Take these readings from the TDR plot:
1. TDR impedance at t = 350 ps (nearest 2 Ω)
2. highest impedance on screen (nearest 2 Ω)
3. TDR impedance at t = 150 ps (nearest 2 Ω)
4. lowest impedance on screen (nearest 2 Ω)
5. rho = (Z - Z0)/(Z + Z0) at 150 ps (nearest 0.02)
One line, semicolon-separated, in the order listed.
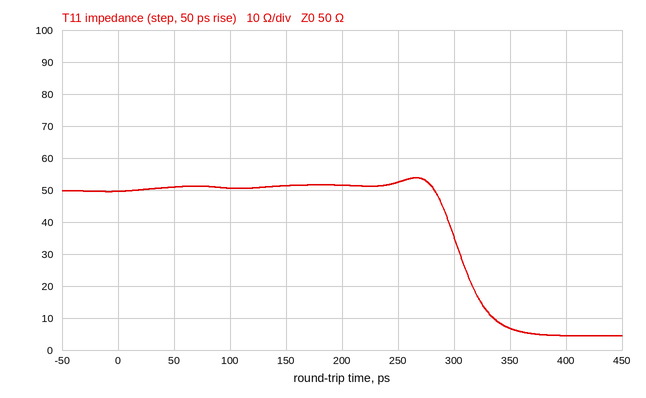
6 Ω; 54 Ω; 52 Ω; 4 Ω; +0.02
